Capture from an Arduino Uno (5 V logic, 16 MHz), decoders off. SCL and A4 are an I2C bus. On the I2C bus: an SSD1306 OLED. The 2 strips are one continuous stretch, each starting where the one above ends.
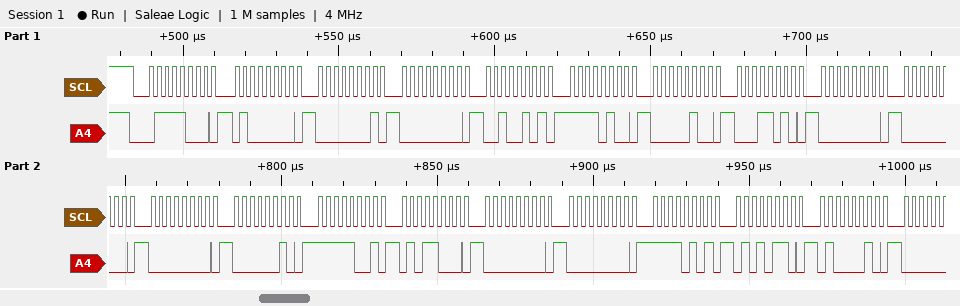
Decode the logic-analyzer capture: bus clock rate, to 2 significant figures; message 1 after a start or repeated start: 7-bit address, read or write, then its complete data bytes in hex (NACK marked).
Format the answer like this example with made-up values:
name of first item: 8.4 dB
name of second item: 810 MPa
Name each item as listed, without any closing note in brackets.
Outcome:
bus clock rate, to 2 significant figures: 400 kHz
message 1 after a start or repeated start: 7-bit address, read or write, then its complete data bytes in hex: 0x3C write: 40 01 00 25 F4 04 1A 00 00 00 02 F9 58 00 00 F5 56 42
